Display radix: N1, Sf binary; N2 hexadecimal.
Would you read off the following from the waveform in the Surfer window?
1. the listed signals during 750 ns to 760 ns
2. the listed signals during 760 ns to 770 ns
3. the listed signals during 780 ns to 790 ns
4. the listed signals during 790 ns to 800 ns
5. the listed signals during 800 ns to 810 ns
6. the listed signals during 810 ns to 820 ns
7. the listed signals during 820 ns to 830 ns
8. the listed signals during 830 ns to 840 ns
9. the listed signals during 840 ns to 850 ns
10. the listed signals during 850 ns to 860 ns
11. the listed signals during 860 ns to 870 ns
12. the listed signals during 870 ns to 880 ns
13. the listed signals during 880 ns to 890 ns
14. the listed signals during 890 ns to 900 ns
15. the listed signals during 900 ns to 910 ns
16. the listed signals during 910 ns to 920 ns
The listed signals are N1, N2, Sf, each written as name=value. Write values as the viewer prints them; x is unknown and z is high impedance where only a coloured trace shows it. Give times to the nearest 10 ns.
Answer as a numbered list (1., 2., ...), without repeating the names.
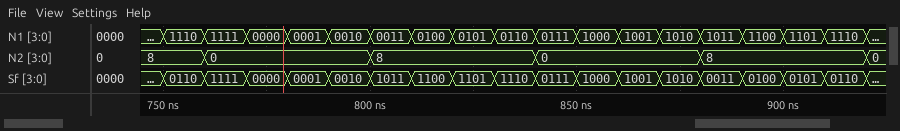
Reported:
1. N1=1110, N2=8, Sf=0110
2. N1=1111, N2=0, Sf=1111
3. N1=0001, N2=0, Sf=0001
4. N1=0010, N2=0, Sf=0010
5. N1=0011, N2=8, Sf=1011
6. N1=0100, N2=8, Sf=1100
7. N1=0101, N2=8, Sf=1101
8. N1=0110, N2=8, Sf=1110
9. N1=0111, N2=0, Sf=0111
10. N1=1000, N2=0, Sf=1000
11. N1=1001, N2=0, Sf=1001
12. N1=1010, N2=0, Sf=1010
13. N1=1011, N2=8, Sf=0011
14. N1=1100, N2=8, Sf=0100
15. N1=1101, N2=8, Sf=0101
16. N1=1110, N2=8, Sf=0110
